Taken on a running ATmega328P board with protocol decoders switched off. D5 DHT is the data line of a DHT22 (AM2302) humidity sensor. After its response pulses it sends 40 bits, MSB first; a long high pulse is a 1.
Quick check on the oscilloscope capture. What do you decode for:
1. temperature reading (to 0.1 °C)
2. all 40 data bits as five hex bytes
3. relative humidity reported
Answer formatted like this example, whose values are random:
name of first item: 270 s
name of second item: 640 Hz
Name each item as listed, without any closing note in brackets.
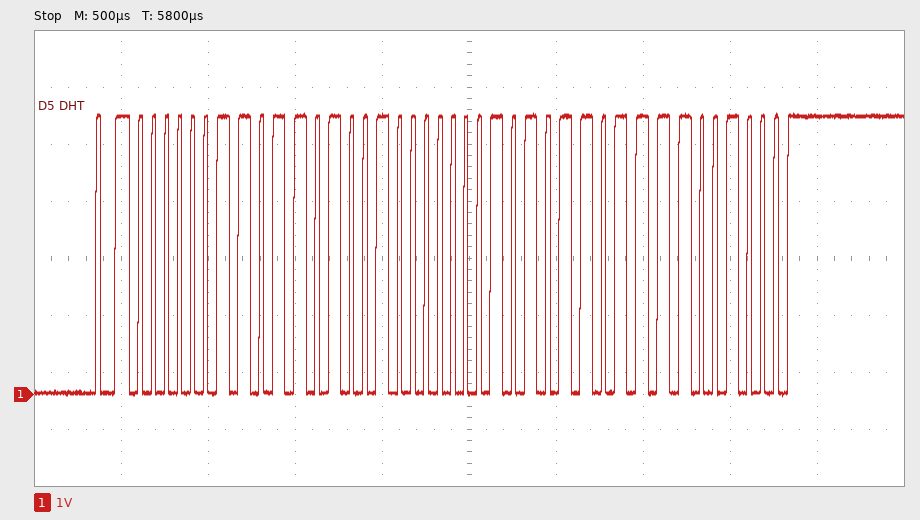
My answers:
temperature reading: 34.7 °C
all 40 data bits as five hex bytes: 03 69 01 5B C8
relative humidity reported: 87.3 %
